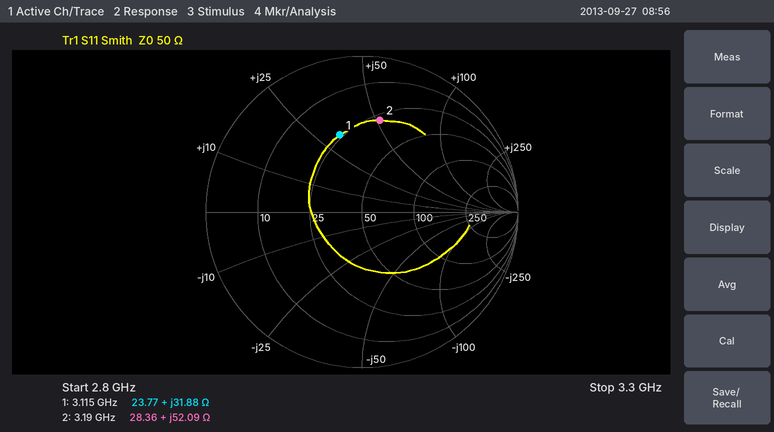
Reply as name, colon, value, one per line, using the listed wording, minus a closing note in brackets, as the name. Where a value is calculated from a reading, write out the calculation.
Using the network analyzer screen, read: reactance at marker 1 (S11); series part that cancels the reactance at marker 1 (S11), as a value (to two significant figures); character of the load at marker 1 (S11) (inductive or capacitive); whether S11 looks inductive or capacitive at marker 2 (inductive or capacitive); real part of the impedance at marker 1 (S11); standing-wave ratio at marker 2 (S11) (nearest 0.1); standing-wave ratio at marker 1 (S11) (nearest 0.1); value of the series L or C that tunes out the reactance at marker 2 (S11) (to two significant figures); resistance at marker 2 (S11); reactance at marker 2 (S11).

reactance at marker 1: +31.88 Ω
series part that cancels the reactance at marker 1 (S11), as a value: C = 1/(2π × 3.115 GHz × 31.88 Ω) ≈ 1.6 pF
character of the load at marker 1 (S11): inductive
whether S11 looks inductive or capacitive at marker 2: inductive
real part of the impedance at marker 1: 23.77 Ω
standing-wave ratio at marker 2 (S11): 4.0
standing-wave ratio at marker 1 (S11): 3.1
value of the series L or C that tunes out the reactance at marker 2 (S11): C = 1/(2π × 3.19 GHz × 52.09 Ω) ≈ 958 fF, so 960 fF to two significant figures
resistance at marker 2: 28.36 Ω
reactance at marker 2: +52.09 Ω
